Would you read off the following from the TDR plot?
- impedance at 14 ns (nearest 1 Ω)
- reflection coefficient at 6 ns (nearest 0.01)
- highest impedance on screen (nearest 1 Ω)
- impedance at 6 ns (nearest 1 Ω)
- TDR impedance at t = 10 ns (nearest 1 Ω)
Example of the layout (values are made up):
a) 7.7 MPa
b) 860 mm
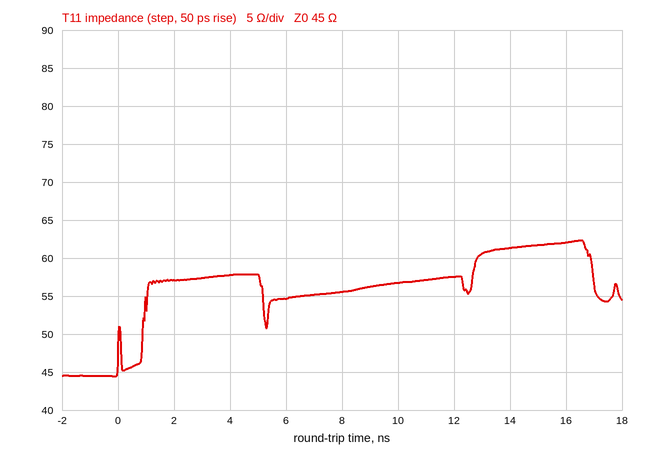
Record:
a) 61 Ω
b) +0.10
c) 62 Ω
d) 55 Ω
e) 57 Ω
